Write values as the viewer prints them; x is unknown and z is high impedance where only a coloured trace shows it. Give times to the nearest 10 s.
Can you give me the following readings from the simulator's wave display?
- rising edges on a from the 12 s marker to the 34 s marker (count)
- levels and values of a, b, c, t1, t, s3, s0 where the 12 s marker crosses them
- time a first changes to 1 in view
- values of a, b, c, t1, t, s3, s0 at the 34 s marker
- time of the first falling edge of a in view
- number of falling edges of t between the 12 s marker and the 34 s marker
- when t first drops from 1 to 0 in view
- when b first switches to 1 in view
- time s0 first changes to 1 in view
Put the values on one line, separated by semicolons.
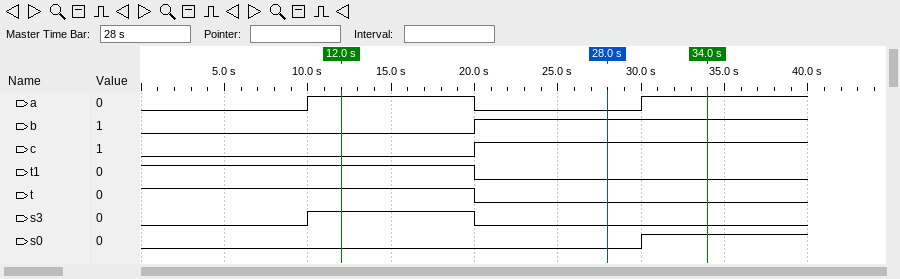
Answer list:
1; a=1, b=0, c=0, t1=1, t=1, s3=1, s0=0; 10 s; a=1, b=1, c=1, t1=0, t=0, s3=0, s0=1; 20 s; 1; 20 s; 20 s; 30 s
